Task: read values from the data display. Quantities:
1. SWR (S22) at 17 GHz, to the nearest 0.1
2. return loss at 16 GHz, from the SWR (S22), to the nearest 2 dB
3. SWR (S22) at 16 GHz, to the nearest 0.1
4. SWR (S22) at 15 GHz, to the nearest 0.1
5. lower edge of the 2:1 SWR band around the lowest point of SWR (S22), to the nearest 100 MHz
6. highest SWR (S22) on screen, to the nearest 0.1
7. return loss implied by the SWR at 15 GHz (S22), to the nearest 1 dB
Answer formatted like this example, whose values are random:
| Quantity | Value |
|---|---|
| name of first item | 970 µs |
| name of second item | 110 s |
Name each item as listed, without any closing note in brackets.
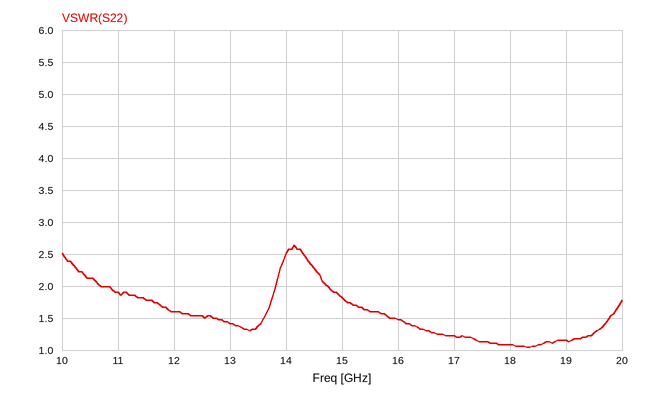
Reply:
| Quantity | Value |
|---|---|
| SWR (S22) at 17 GHz, to the nearest 0.1 | 1.2 |
| return loss at 16 GHz, from the SWR (S22), to the nearest 2 dB | 14 dB |
| SWR (S22) at 16 GHz, to the nearest 0.1 | 1.5 |
| SWR (S22) at 15 GHz, to the nearest 0.1 | 1.8 |
| lower edge of the 2:1 SWR band around the lowest point of SWR (S22), to the nearest 100 MHz | 14.7 GHz |
| highest SWR (S22) on screen, to the nearest 0.1 | 2.6 |
| return loss implied by the SWR at 15 GHz (S22), to the nearest 1 dB | 11 dB |
